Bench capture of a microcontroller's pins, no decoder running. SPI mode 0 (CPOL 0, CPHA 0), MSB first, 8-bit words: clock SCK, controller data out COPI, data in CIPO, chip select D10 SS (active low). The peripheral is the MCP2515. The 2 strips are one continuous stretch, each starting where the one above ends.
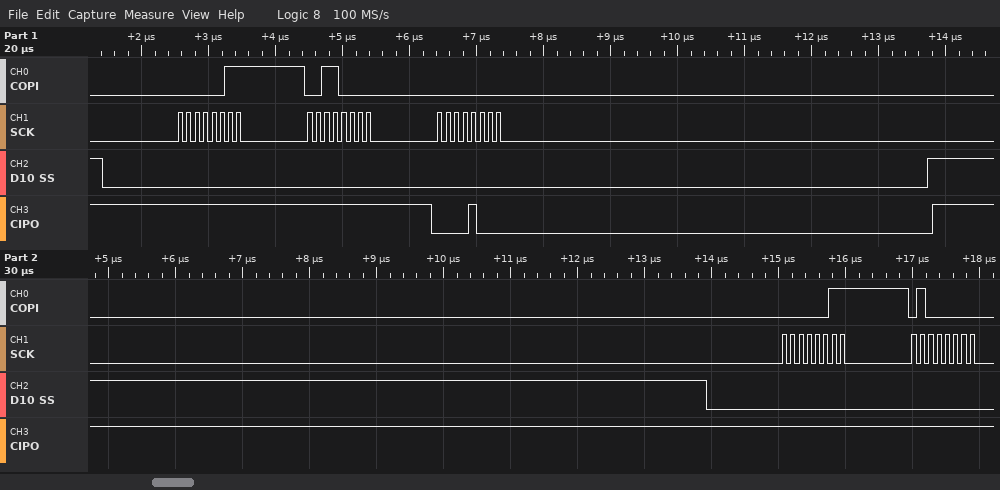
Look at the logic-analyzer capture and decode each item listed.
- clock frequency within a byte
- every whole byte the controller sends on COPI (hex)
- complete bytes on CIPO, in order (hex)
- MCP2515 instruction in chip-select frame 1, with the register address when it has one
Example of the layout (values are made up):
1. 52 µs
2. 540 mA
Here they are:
1. 8 MHz
2. 03 30 00 03 40
3. FF FF 08 FF FF
4. READ 0x30
